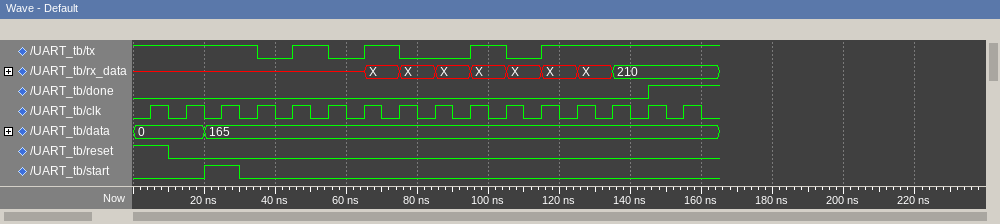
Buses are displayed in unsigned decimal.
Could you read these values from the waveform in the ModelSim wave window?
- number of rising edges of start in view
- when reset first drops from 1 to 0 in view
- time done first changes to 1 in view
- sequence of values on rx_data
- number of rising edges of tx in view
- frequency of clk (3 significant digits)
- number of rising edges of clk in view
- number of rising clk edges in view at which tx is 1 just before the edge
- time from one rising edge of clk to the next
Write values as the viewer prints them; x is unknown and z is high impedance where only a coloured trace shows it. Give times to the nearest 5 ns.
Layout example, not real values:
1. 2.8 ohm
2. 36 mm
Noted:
1. 1
2. 10 ns
3. 145 ns
4. x, X, X, X, X, X, X, X, 210
5. 4
6. 100 MHz
7. 16
8. 11
9. 10 ns
